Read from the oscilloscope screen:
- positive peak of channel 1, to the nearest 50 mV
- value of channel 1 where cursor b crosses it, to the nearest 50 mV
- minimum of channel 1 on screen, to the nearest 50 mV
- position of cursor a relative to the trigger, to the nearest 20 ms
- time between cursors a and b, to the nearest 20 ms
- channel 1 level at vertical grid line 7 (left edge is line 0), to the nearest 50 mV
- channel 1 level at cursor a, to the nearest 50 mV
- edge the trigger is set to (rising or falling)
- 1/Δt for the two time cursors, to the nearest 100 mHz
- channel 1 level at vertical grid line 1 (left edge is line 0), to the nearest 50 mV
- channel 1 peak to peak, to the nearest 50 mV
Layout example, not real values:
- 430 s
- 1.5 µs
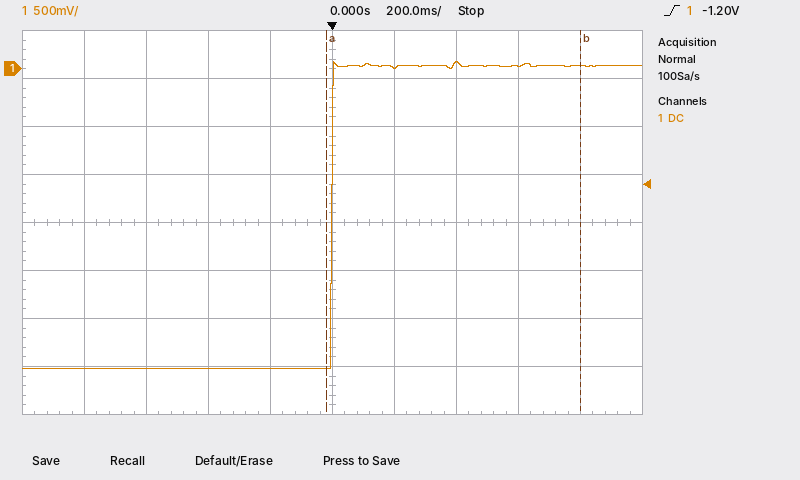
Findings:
- 100 mV
- 50 mV
- -3.10 V
- -20 ms
- 820 ms
- 50 mV
- -3.10 V
- rising
- 1.2 Hz
- -3.10 V
- 3.20 V
